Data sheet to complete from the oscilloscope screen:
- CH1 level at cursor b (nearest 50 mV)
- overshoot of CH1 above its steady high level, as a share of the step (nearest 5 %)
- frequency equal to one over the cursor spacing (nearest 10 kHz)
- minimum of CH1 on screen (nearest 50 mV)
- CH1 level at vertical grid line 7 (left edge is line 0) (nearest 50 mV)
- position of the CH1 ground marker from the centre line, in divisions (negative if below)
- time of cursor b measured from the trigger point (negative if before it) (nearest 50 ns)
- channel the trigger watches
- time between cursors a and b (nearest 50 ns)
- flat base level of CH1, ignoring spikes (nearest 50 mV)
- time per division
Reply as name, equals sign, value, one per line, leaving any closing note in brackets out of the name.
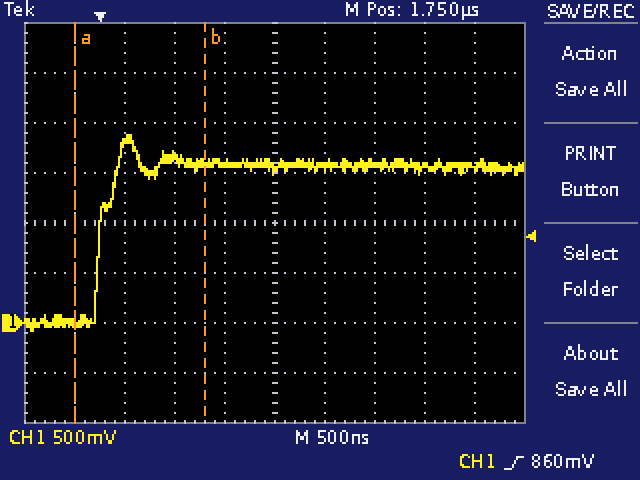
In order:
CH1 level at cursor b = 1.60 V
overshoot of CH1 above its steady high level, as a share of the step = 20 %
frequency equal to one over the cursor spacing = 770 kHz
minimum of CH1 on screen = -100 mV
CH1 level at vertical grid line 7 (left edge is line 0) = 1.60 V
position of the CH1 ground marker from the centre line, in divisions = -2.0 div
time of cursor b measured from the trigger point (negative if before it) = +1.05 µs
channel the trigger watches = CH1
time between cursors a and b = 1.30 µs
flat base level of CH1, ignoring spikes = 0 mV
time per division = 500 ns
